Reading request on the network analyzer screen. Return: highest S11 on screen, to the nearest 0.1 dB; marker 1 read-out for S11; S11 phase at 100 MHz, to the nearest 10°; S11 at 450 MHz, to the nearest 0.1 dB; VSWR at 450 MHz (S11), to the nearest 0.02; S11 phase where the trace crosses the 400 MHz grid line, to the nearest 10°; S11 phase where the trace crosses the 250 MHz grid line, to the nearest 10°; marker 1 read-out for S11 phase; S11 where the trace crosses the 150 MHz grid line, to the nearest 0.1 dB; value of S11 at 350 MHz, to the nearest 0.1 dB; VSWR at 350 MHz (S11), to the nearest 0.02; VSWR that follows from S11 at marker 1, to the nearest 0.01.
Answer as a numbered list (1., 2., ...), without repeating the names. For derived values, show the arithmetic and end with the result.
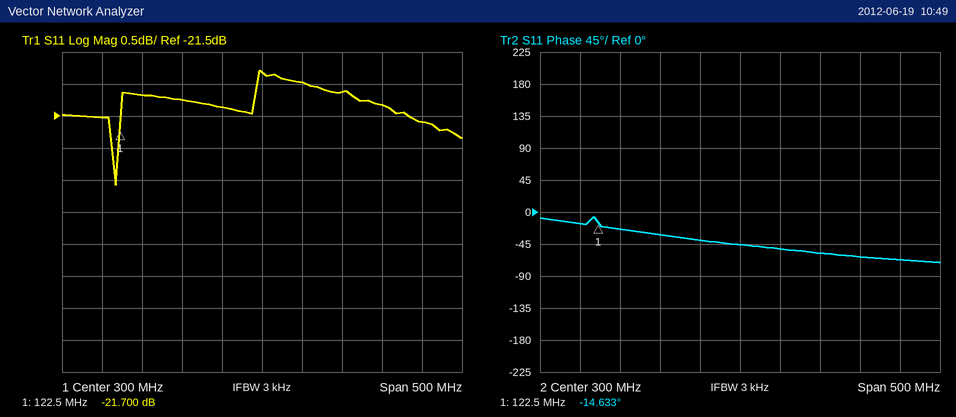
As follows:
1. -20.8 dB
2. -21.700 dB
3. -20°
4. -21.3 dB
5. |Γ| = 10^(-21.3/20) = 0.0861; VSWR = (1 + 0.0861)/(1 − 0.0861) ≈ 1.19, so 1.18 to the nearest 0.02
6. -60°
7. -40°
8. -14.633°
9. -21.2 dB
10. -21.0 dB
11. |Γ| = 10^(-21/20) = 0.0891; VSWR = (1 + 0.0891)/(1 − 0.0891) ≈ 1.20
12. (1 + 0.0822)/(1 − 0.0822) ≈ 1.18
